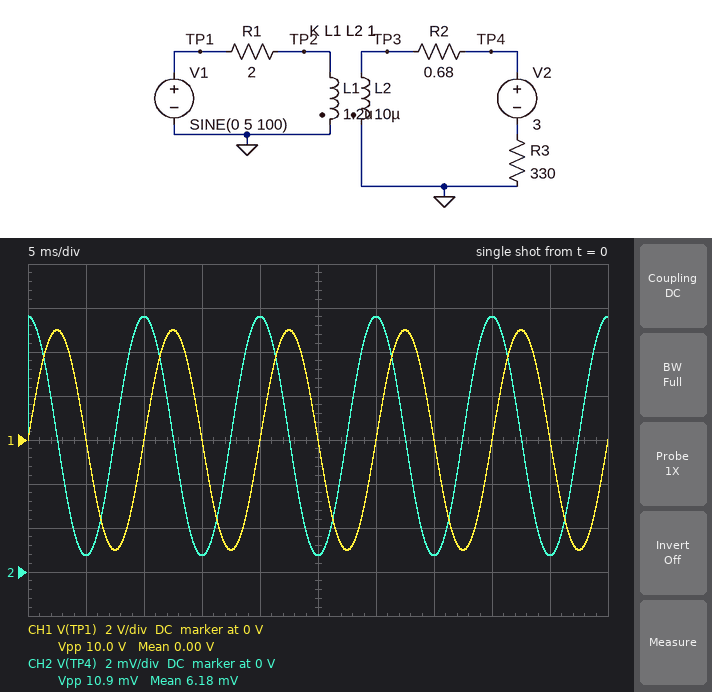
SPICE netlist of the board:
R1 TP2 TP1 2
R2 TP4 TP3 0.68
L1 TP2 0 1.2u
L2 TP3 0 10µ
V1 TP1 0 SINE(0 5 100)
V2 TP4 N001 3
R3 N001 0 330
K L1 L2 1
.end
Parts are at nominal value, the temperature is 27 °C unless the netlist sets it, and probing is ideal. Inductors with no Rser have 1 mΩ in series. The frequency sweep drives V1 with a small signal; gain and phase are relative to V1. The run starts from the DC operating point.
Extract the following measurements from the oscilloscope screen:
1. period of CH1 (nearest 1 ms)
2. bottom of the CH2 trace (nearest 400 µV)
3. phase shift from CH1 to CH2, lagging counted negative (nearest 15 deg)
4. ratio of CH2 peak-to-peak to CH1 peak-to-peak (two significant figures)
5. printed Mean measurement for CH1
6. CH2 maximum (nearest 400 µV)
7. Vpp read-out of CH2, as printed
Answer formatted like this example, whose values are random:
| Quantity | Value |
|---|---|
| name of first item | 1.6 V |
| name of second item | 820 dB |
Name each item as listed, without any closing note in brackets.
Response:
| Quantity | Value |
|---|---|
| period of CH1 | 10 ms |
| bottom of the CH2 trace | 800 µV |
| phase shift from CH1 to CH2, lagging counted negative | 90 deg |
| ratio of CH2 peak-to-peak to CH1 peak-to-peak | 0.0011 |
| printed Mean measurement for CH1 | 0.00 V |
| CH2 maximum | 11.6 mV |
| Vpp read-out of CH2, as printed | 10.9 mV |
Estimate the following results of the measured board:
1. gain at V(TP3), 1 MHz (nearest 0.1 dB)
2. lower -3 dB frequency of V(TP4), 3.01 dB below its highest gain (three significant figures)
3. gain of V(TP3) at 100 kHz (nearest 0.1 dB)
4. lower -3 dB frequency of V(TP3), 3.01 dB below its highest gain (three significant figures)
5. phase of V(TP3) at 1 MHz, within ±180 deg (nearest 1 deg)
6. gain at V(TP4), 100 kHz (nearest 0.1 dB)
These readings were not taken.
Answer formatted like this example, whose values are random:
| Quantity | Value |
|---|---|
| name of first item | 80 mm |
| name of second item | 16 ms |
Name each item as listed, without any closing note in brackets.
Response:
| Quantity | Value |
|---|---|
| gain at V(TP3), 1 MHz | 8.5 dB |
| lower -3 dB frequency of V(TP4), 3.01 dB below its highest gain | 253 kHz |
| gain of V(TP3) at 100 kHz | 0.1 dB |
| lower -3 dB frequency of V(TP3), 3.01 dB below its highest gain | 253 kHz |
| phase of V(TP3) at 1 MHz, within ±180 deg | 14 deg |
| gain at V(TP4), 100 kHz | 0.1 dB |
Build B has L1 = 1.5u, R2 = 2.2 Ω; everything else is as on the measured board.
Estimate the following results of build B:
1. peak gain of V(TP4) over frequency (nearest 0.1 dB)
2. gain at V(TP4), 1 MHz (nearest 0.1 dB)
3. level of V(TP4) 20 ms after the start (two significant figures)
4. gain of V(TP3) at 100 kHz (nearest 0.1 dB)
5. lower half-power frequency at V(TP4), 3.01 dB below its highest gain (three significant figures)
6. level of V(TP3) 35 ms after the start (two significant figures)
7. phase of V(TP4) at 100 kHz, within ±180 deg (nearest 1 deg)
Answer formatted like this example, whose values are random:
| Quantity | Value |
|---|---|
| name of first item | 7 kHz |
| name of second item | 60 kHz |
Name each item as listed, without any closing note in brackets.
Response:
| Quantity | Value |
|---|---|
| peak gain of V(TP4) over frequency | 7.8 dB |
| gain at V(TP4), 1 MHz | 7.7 dB |
| level of V(TP4) 20 ms after the start | 26 mV |
| gain of V(TP3) at 100 kHz | 0.8 dB |
| lower half-power frequency at V(TP4), 3.01 dB below its highest gain | 204 kHz |
| level of V(TP3) 35 ms after the start | -6.1 mV |
| phase of V(TP4) at 100 kHz, within ±180 deg | 64 deg |
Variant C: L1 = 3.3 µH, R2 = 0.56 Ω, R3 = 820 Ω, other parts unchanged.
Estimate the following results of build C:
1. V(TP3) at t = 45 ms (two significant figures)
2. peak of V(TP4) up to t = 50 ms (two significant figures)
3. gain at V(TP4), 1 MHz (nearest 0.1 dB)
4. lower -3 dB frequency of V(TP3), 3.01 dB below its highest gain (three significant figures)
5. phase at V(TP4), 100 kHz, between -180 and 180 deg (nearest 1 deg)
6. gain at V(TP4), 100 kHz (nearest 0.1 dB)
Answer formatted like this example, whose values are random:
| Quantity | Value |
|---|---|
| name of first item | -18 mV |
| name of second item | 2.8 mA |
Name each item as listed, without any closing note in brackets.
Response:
| Quantity | Value |
|---|---|
| V(TP3) at t = 45 ms | -9.0 mV |
| peak of V(TP4) up to t = 50 ms | 11 mV |
| gain at V(TP4), 1 MHz | 4.7 dB |
| lower -3 dB frequency of V(TP3), 3.01 dB below its highest gain | 95.8 kHz |
| phase at V(TP4), 100 kHz, between -180 and 180 deg | 44 deg |
| gain at V(TP4), 100 kHz | 1.9 dB |
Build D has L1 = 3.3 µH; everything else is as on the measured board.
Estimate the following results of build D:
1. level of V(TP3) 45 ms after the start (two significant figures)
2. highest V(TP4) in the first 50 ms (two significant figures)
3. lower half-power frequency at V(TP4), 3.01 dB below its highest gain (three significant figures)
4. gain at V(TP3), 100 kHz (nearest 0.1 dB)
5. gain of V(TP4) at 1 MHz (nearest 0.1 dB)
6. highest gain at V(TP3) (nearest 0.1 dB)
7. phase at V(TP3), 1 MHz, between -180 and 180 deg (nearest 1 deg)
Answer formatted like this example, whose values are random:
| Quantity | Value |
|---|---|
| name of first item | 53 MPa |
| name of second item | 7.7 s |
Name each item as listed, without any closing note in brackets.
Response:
| Quantity | Value |
|---|---|
| level of V(TP3) 45 ms after the start | -9.0 mV |
| highest V(TP4) in the first 50 ms | 15 mV |
| lower half-power frequency at V(TP4), 3.01 dB below its highest gain | 94.8 kHz |
| gain at V(TP3), 100 kHz | 1.9 dB |
| gain of V(TP4) at 1 MHz | 4.6 dB |
| highest gain at V(TP3) | 4.7 dB |
| phase at V(TP3), 1 MHz, between -180 and 180 deg | 5 deg |
